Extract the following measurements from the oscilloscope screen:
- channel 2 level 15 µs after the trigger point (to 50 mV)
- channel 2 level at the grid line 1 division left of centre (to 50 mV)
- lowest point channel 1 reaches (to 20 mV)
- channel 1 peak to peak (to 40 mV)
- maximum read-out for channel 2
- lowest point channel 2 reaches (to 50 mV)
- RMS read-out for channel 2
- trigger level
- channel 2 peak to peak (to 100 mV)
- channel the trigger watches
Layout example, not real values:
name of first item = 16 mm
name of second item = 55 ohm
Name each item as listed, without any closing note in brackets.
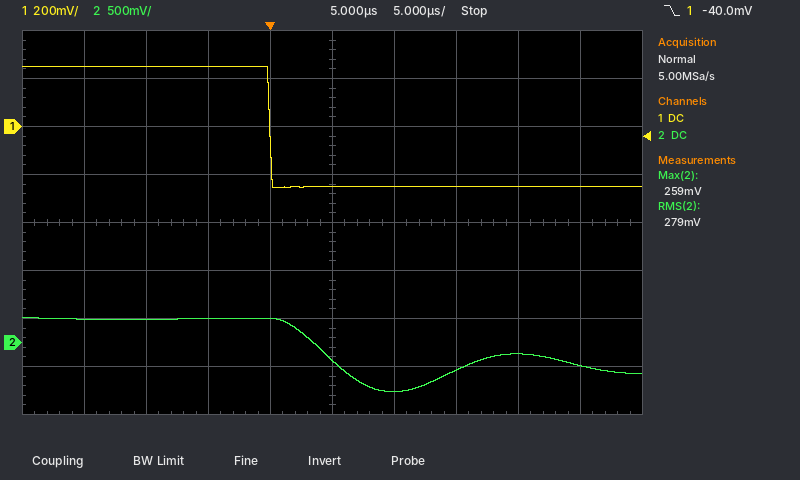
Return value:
channel 2 level 15 µs after the trigger point = -300 mV
channel 2 level at the grid line 1 division left of centre = 250 mV
lowest point channel 1 reaches = -260 mV
channel 1 peak to peak = 520 mV
maximum read-out for channel 2 = 259 mV
lowest point channel 2 reaches = -500 mV
RMS read-out for channel 2 = 279 mV
trigger level = -40.0 mV
channel 2 peak to peak = 800 mV
channel the trigger watches = channel 1
